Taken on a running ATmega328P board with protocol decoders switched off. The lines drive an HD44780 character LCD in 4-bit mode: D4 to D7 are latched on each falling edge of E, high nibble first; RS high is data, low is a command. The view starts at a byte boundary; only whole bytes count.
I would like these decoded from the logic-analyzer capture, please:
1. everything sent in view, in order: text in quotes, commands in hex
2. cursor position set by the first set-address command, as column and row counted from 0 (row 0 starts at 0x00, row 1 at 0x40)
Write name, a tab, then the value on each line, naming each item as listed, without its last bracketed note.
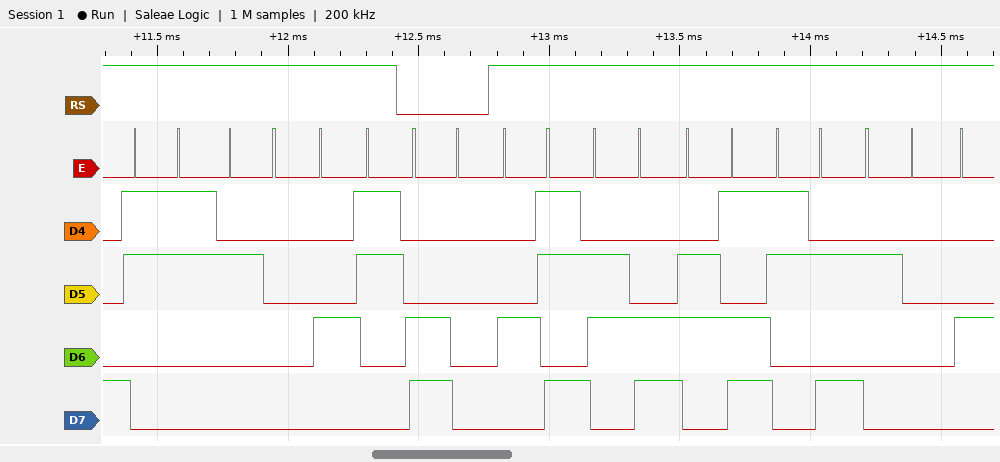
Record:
everything sent in view, in order: text in quotes, commands in hex	"3 C" 0xC0 "Klm: "
cursor position set by the first set-address command, as column and row counted from 0	column 0, row 1
